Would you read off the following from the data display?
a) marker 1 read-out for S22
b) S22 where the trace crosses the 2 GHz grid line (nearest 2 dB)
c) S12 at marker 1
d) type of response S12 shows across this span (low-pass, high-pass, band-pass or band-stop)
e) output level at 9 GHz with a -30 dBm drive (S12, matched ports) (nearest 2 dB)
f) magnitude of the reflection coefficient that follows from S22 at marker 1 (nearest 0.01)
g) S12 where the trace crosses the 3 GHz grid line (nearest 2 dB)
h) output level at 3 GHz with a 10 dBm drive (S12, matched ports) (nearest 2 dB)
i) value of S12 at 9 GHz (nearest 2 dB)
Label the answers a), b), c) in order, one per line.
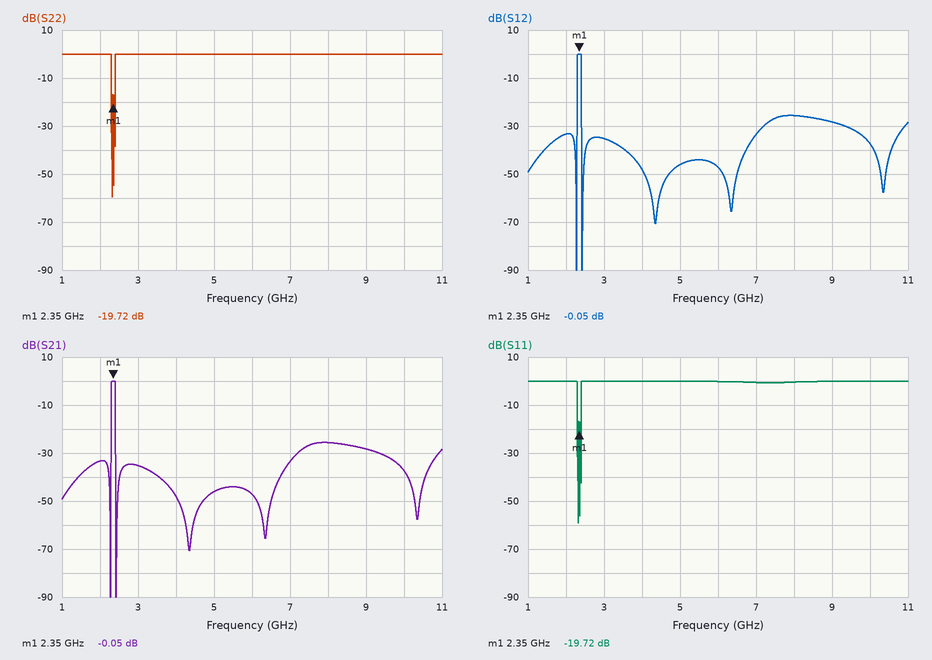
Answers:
a) -19.72 dB
b) 0 dB
c) -0.05 dB
d) band-pass
e) -58 dBm
f) 0.10
g) -36 dB
h) -26 dBm
i) -28 dB
